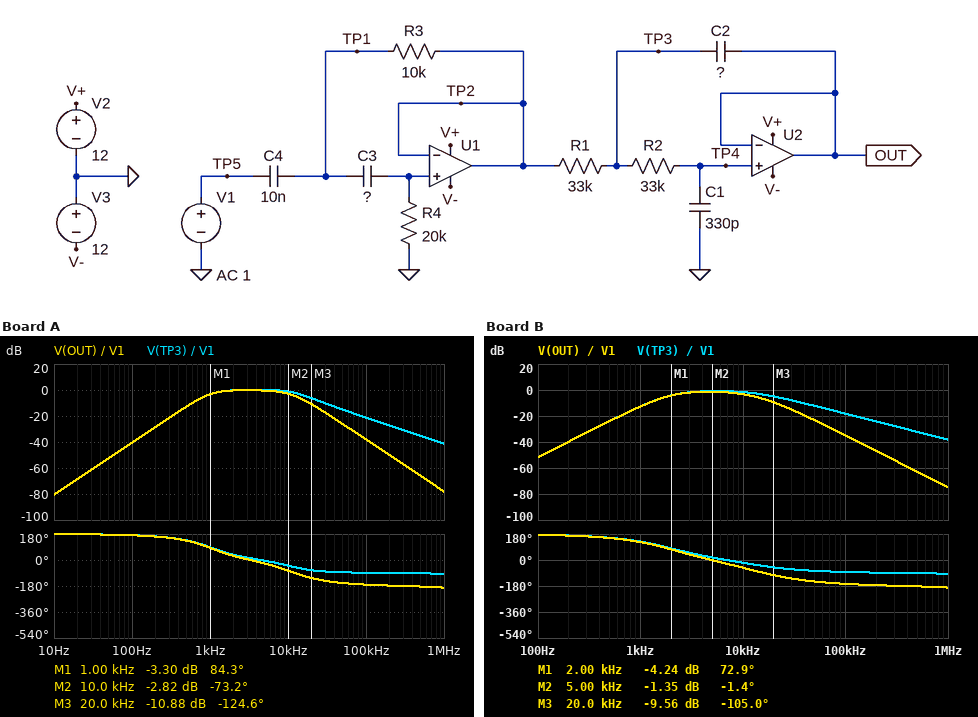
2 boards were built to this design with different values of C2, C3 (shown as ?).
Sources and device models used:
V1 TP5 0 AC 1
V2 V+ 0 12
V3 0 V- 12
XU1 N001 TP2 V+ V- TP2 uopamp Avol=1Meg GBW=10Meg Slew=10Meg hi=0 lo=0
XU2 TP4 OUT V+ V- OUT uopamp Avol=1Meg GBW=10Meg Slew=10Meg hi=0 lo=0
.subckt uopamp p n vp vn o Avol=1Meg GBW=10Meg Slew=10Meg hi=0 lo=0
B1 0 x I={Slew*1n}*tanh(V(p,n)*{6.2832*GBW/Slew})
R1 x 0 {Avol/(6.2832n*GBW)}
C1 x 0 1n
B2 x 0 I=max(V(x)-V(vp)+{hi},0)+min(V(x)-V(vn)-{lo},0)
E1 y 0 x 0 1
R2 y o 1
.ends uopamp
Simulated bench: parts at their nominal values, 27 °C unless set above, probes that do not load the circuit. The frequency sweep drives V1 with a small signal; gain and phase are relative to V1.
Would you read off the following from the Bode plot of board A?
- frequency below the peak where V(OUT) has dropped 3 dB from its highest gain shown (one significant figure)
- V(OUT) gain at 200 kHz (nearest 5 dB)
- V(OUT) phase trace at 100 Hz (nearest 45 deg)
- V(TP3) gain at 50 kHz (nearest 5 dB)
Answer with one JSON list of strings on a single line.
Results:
["1 kHz", "-50 dB", "180 deg", "-15 dB"]
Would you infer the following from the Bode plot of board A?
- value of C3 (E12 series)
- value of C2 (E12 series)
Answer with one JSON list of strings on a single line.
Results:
["12 nF", "560 pF"]
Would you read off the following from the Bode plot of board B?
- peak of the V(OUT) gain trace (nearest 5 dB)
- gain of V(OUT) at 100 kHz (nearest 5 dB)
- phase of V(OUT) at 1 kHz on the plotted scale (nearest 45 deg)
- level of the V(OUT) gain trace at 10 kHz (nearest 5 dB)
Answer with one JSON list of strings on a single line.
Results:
["0 dB", "-35 dB", "135 deg", "-5 dB"]
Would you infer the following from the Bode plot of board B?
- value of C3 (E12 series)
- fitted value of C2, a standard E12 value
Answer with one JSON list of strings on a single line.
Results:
["3.3 nF", "390 pF"]
